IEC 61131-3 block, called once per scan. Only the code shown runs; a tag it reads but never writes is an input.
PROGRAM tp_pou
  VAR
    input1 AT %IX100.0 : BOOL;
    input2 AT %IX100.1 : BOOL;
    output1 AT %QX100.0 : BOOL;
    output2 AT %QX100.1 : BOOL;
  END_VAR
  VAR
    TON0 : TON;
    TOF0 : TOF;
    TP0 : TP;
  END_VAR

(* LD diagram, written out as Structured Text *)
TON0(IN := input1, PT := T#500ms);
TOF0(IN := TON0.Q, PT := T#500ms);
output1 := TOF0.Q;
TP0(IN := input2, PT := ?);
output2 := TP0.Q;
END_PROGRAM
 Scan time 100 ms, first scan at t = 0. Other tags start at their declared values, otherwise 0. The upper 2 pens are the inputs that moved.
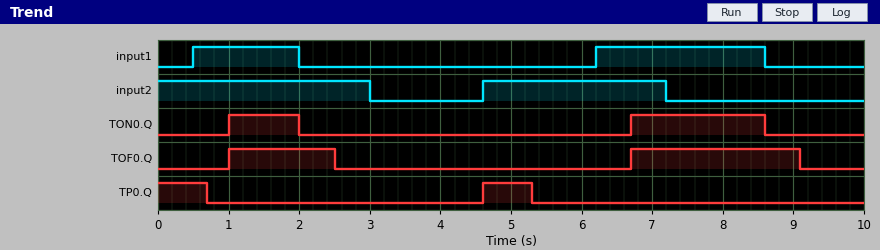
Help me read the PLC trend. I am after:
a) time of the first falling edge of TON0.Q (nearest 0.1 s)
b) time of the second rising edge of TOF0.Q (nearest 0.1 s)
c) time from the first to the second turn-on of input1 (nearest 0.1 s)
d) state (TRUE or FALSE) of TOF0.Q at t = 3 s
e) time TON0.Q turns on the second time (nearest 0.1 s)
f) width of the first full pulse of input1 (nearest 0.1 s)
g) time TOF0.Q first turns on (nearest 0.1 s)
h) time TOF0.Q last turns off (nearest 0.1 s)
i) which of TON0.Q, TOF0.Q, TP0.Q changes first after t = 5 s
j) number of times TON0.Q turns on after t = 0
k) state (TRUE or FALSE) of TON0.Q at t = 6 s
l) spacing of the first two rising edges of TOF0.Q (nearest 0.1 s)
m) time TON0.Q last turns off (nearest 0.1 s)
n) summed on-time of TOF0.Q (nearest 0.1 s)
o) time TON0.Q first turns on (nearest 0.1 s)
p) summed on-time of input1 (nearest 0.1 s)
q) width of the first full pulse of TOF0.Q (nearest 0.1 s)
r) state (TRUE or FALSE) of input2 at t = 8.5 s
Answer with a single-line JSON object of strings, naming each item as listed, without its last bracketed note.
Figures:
{"time of the first falling edge of TON0.Q": "2.0 s", "time of the second rising edge of TOF0.Q": "6.7 s", "time from the first to the second turn-on of input1": "5.7 s", "state (TRUE or FALSE) of TOF0.Q at t = 3 s": "FALSE", "time TON0.Q turns on the second time": "6.7 s", "width of the first full pulse of input1": "1.5 s", "time TOF0.Q first turns on": "1.0 s", "time TOF0.Q last turns off": "9.1 s", "which of TON0.Q, TOF0.Q, TP0.Q changes first after t = 5 s": "TP0.Q", "number of times TON0.Q turns on after t = 0": "2", "state (TRUE or FALSE) of TON0.Q at t = 6 s": "FALSE", "spacing of the first two rising edges of TOF0.Q": "5.7 s", "time TON0.Q last turns off": "8.6 s", "summed on-time of TOF0.Q": "3.9 s", "time TON0.Q first turns on": "1.0 s", "summed on-time of input1": "3.9 s", "width of the first full pulse of TOF0.Q": "1.5 s", "state (TRUE or FALSE) of input2 at t = 8.5 s": "FALSE"}
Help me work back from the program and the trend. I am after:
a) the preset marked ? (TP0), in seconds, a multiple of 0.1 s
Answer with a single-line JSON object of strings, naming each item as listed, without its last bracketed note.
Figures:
{"the preset marked ? (TP0), in seconds, a multiple of 0.1 s": "0.7 s"}
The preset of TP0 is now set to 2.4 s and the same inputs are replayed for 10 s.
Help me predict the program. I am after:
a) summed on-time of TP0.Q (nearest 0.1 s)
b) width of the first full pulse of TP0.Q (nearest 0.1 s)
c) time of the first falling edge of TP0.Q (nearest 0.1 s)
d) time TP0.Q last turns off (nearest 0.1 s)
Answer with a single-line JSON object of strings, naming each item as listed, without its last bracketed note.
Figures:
{"summed on-time of TP0.Q": "4.8 s", "width of the first full pulse of TP0.Q": "2.4 s", "time of the first falling edge of TP0.Q": "2.4 s", "time TP0.Q last turns off": "7.0 s"}
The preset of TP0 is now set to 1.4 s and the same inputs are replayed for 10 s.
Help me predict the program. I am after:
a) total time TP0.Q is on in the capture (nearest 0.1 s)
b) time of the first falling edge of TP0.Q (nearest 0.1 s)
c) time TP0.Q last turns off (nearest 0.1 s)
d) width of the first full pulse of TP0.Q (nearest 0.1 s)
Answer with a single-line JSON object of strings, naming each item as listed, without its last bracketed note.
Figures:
{"total time TP0.Q is on in the capture": "2.8 s", "time of the first falling edge of TP0.Q": "1.4 s", "time TP0.Q last turns off": "6.0 s", "width of the first full pulse of TP0.Q": "1.4 s"}
